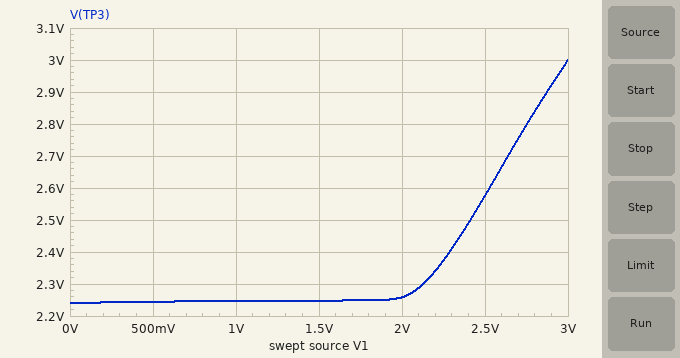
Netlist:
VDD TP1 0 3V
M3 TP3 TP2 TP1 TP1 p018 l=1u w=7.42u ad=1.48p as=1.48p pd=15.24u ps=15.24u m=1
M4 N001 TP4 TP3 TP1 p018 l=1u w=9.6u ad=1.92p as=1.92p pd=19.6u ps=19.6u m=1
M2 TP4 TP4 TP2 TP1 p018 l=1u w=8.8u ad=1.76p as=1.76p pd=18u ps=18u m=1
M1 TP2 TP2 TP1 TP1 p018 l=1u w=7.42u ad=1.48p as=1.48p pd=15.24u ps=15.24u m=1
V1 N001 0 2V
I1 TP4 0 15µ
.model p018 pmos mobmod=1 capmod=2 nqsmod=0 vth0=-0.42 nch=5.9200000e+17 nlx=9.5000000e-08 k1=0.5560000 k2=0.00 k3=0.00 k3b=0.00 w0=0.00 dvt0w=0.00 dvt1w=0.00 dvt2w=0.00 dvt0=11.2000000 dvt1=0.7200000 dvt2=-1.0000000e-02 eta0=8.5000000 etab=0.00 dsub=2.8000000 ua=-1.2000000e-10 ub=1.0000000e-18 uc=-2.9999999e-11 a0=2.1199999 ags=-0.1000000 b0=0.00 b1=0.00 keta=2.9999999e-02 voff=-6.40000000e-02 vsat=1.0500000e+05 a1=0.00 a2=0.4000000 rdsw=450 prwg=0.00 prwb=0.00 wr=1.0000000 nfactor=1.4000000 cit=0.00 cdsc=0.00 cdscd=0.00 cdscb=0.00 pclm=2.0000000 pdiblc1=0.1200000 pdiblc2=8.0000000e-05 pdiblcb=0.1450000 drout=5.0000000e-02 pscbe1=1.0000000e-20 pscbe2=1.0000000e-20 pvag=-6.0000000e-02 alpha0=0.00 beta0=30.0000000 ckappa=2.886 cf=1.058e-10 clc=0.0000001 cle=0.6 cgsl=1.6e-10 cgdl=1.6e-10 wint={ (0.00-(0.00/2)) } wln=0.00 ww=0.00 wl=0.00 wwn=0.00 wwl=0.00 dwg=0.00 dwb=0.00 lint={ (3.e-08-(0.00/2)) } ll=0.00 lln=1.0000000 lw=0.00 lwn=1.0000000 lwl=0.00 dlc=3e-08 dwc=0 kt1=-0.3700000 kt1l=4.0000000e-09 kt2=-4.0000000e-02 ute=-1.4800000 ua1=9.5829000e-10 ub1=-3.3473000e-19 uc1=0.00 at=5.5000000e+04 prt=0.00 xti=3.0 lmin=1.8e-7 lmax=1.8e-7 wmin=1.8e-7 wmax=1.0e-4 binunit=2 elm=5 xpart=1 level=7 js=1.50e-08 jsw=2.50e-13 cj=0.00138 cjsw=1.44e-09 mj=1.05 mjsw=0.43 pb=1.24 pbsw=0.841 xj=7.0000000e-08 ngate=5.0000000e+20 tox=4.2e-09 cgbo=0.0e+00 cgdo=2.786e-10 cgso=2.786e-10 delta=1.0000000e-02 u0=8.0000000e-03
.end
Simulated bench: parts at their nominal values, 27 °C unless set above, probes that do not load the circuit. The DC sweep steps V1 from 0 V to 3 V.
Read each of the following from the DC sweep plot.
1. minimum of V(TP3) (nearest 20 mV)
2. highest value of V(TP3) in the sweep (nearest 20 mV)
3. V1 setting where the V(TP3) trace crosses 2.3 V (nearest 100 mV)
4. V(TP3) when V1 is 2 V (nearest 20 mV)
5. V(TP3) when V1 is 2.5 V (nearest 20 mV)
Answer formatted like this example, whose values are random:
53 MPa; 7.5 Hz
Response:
2.24 V; 3.00 V; 2.1 V; 2.26 V; 2.58 V
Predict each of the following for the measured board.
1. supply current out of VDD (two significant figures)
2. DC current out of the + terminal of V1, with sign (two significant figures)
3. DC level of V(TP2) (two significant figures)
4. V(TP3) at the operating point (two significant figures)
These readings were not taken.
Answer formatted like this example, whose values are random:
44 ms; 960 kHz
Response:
30 µA; -15 µA; 2.3 V; 2.3 V
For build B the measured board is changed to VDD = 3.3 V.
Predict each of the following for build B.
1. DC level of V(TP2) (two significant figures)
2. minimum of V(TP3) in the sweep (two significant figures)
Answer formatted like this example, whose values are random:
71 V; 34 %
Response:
2.6 V; 2.5 V
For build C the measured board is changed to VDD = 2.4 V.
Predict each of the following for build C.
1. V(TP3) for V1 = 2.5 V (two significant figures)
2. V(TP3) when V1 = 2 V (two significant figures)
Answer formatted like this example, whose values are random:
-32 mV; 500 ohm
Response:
2.5 V; 2.1 V
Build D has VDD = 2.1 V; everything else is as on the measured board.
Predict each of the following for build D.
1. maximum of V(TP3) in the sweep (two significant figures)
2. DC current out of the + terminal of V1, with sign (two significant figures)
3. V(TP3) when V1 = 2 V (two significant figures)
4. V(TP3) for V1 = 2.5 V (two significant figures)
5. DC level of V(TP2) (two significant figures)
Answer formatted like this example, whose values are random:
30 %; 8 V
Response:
2.8 V; -6.5 µA; 2.0 V; 2.4 V; 1.4 V
